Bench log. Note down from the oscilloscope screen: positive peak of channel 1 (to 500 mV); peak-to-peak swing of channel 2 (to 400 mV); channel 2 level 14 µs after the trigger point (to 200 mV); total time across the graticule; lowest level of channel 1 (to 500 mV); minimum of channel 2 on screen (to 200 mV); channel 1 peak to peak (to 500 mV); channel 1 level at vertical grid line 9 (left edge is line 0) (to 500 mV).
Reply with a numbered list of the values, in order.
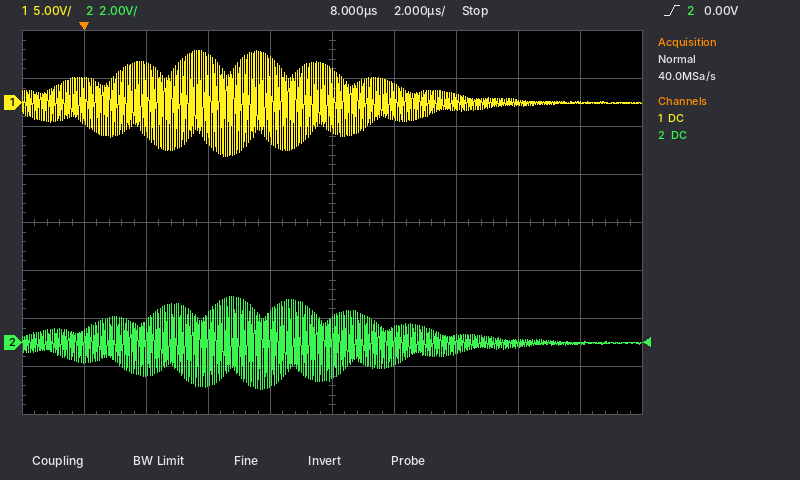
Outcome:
1. 5.5 V
2. 4.0 V
3. 0.0 V
4. 20 µs
5. -5.5 V
6. -2.0 V
7. 11.0 V
8. 0.0 V
